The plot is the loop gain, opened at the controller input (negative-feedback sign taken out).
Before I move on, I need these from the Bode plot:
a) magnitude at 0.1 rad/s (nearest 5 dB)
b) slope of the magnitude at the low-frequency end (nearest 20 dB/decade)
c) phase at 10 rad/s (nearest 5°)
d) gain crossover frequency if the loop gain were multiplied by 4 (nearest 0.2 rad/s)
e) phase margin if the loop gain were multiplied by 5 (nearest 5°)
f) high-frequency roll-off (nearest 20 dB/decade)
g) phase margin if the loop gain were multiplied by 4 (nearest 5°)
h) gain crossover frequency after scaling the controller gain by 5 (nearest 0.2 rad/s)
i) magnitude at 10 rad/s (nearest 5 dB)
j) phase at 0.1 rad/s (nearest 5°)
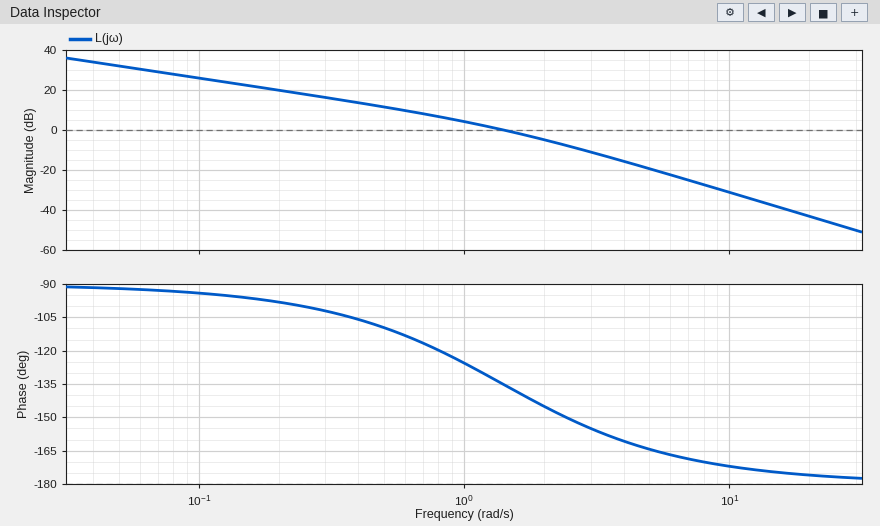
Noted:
25 dB
-20 dB/decade
-170°
3.2 rad/s
20°
-40 dB/decade
25°
3.6 rad/s
-30 dB
-95°
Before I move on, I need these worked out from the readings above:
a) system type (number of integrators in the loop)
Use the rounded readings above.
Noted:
1
